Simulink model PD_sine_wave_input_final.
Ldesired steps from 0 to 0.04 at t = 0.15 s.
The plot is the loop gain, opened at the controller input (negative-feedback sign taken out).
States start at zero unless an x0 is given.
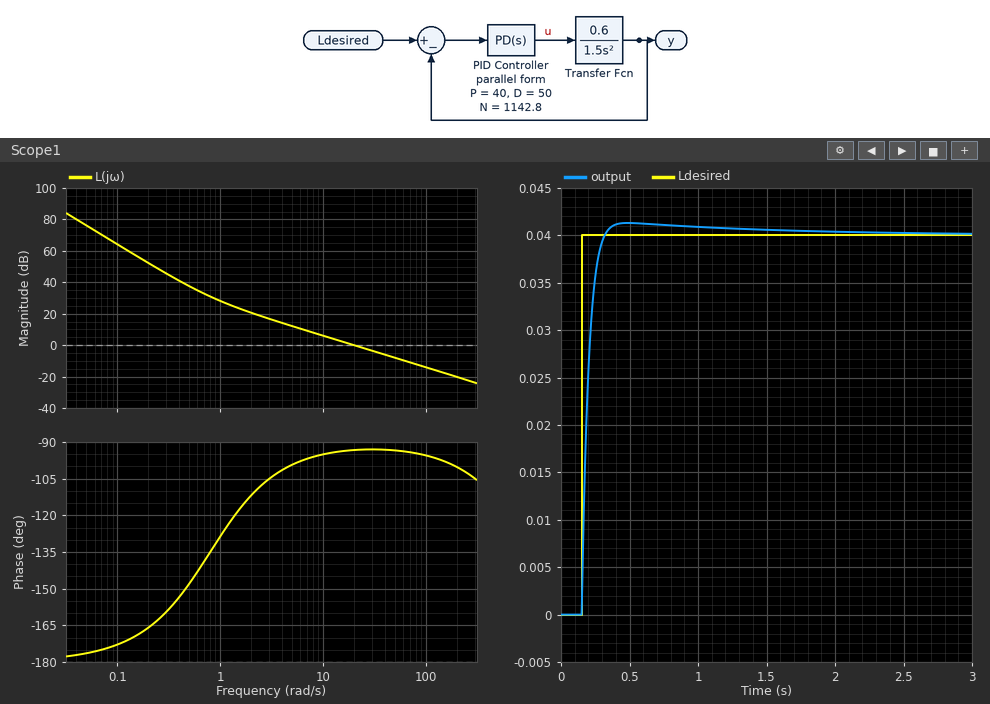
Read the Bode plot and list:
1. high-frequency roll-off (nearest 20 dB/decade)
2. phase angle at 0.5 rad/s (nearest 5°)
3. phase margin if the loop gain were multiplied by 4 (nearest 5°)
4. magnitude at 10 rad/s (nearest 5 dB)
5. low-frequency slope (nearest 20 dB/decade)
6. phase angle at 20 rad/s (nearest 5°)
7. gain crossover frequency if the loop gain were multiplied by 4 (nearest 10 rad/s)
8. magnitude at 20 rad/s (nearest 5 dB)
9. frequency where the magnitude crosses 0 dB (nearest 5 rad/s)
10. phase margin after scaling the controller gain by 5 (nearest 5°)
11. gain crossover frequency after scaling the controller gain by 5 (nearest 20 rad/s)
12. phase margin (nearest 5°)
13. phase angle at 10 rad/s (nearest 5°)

-20 dB/decade
-150°
85°
5 dB
-40 dB/decade
-95°
80 rad/s
0 dB
20 rad/s
85°
100 rad/s
85°
-95°
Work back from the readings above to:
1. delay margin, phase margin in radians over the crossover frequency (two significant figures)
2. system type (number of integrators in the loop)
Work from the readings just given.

0.074 s
2
